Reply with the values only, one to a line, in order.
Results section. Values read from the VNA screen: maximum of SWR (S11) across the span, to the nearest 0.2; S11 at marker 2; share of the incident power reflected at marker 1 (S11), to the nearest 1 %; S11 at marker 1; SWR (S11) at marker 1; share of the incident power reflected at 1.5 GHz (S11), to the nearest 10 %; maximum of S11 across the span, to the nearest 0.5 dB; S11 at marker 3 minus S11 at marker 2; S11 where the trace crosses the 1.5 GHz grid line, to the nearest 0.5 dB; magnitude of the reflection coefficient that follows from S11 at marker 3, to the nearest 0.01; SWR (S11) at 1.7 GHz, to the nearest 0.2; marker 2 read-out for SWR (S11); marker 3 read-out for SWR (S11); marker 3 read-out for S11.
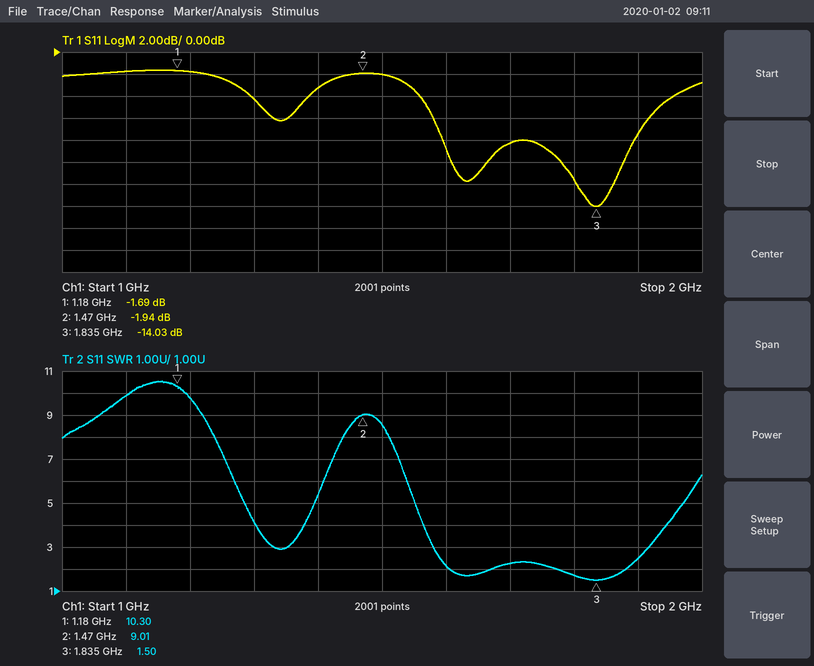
10.6
-1.94 dB
68 %
-1.69 dB
10.30
60 %
-1.5 dB
-12.09 dB
-2.0 dB
0.20
2.2
9.01
1.50
-14.03 dB
